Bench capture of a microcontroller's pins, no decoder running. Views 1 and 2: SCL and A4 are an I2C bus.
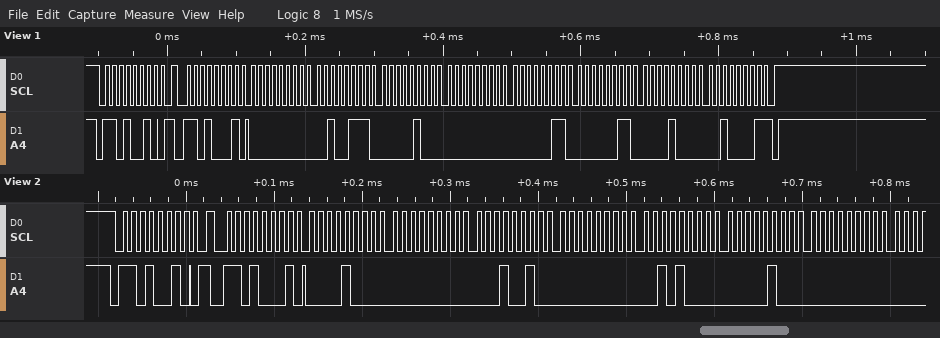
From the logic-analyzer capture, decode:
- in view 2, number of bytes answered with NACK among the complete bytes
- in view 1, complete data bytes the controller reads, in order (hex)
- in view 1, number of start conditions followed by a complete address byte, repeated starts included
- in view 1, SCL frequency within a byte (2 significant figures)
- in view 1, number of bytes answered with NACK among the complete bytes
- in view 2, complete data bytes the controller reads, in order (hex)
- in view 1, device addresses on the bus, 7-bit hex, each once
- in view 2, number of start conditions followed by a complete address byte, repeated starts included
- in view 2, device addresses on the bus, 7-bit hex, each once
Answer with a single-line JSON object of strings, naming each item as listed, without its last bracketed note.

{"in view 2, number of bytes answered with NACK among the complete bytes": "0", "in view 1, complete data bytes the controller reads, in order": "00 27 04 00 03 03 08 21", "in view 1, number of start conditions followed by a complete address byte, repeated starts included": "2", "in view 1, SCL frequency within a byte": "100 kHz", "in view 1, number of bytes answered with NACK among the complete bytes": "1", "in view 2, complete data bytes the controller reads, in order": "08 00 12 00 28 04 00", "in view 1, device addresses on the bus, 7-bit hex, each once": "0x69 0x68", "in view 2, number of start conditions followed by a complete address byte, repeated starts included": "2", "in view 2, device addresses on the bus, 7-bit hex, each once": "0x69 0x68"}
